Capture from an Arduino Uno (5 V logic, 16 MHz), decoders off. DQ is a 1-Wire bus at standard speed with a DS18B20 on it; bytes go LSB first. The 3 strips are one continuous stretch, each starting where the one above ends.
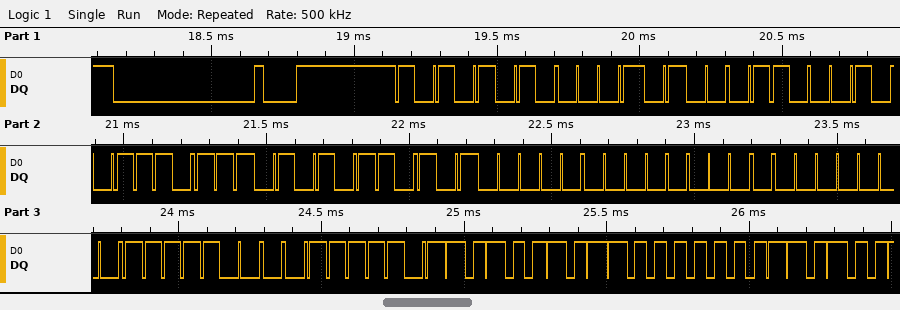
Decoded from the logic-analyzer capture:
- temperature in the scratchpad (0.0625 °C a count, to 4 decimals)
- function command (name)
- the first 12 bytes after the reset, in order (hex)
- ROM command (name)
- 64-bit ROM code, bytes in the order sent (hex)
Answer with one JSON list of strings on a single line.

["26.3125 °C", "Read Scratchpad", "55 28 46 EE 6A 05 00 00 1F BE A5 01", "Match ROM", "28 46 EE 6A 05 00 00 1F"]
